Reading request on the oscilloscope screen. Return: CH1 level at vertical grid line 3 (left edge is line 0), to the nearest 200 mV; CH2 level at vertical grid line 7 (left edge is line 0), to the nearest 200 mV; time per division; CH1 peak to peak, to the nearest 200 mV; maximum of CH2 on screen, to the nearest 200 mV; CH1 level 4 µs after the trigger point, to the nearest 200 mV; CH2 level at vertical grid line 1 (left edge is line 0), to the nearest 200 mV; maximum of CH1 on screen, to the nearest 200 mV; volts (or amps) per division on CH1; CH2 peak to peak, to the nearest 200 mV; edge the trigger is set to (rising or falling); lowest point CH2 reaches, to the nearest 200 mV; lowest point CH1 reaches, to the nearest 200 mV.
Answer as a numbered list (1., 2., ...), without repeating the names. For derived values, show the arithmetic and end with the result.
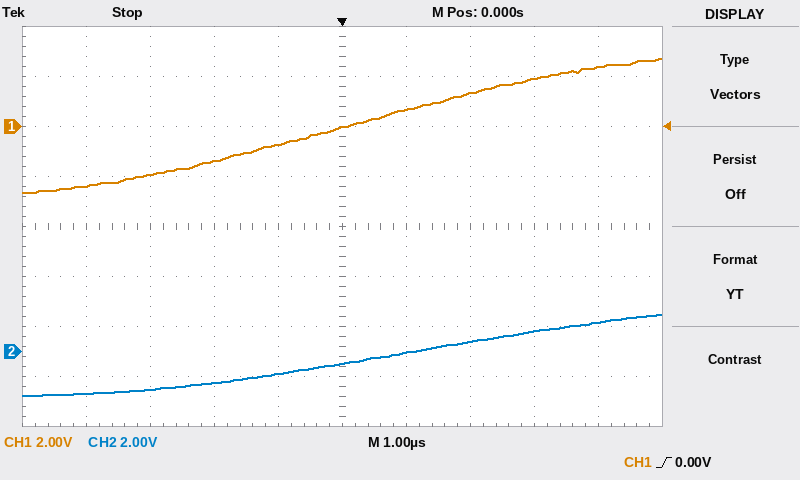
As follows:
1. -1.4 V
2. 400 mV
3. 1 µs
4. 2.8 V − (-2.6 V) = 5.4 V
5. 1.4 V
6. 2.4 V
7. -1.6 V
8. 2.8 V
9. 2 V
10. 1.4 V − (-1.8 V) = 3.2 V
11. rising
12. -1.8 V
13. -2.6 V
